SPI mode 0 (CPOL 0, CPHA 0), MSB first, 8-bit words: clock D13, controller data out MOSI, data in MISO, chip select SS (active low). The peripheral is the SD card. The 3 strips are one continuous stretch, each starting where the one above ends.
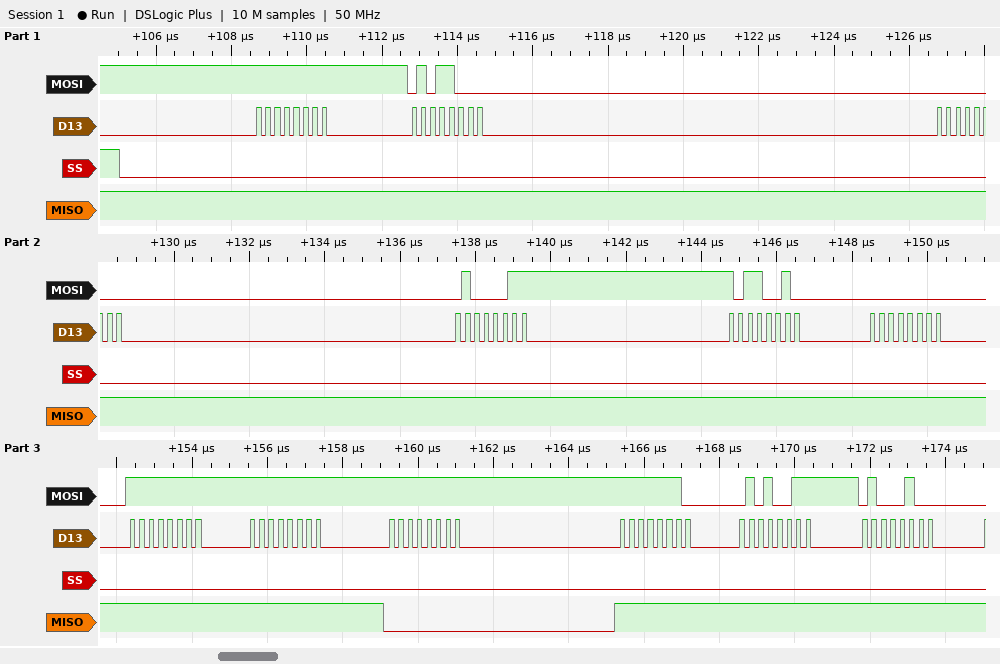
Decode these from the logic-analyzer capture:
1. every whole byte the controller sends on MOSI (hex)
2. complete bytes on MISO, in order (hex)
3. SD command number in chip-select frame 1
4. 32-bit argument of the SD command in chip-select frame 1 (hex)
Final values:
FF 58 00 43 B2 00 FF FF FF FE 53 44
FF FF FF FF FF FF FF FF 00 FF FF FF
CMD24
0x0043B200
